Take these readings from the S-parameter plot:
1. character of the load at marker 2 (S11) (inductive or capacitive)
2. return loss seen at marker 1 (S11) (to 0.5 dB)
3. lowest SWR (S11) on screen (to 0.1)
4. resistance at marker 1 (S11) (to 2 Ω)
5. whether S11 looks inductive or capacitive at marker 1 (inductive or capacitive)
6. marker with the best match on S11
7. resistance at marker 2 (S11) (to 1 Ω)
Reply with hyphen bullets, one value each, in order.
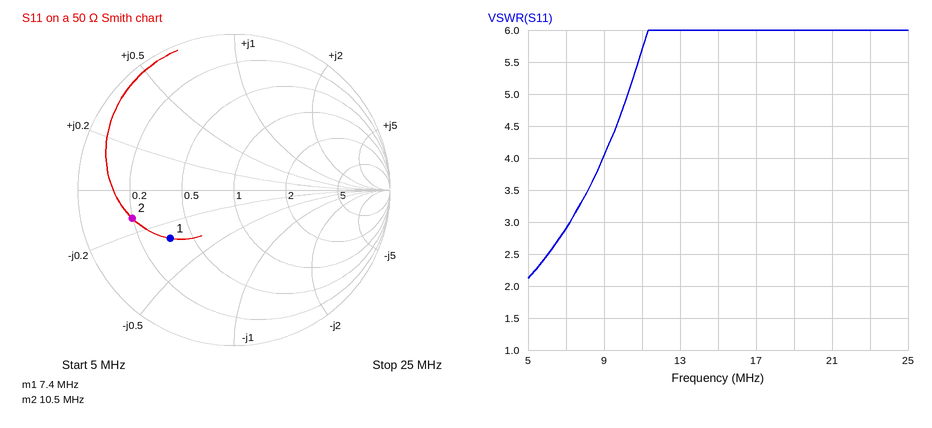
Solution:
- capacitive
- 6.0 dB
- 2.1
- 18 Ω
- capacitive
- marker 1
- 10 Ω
